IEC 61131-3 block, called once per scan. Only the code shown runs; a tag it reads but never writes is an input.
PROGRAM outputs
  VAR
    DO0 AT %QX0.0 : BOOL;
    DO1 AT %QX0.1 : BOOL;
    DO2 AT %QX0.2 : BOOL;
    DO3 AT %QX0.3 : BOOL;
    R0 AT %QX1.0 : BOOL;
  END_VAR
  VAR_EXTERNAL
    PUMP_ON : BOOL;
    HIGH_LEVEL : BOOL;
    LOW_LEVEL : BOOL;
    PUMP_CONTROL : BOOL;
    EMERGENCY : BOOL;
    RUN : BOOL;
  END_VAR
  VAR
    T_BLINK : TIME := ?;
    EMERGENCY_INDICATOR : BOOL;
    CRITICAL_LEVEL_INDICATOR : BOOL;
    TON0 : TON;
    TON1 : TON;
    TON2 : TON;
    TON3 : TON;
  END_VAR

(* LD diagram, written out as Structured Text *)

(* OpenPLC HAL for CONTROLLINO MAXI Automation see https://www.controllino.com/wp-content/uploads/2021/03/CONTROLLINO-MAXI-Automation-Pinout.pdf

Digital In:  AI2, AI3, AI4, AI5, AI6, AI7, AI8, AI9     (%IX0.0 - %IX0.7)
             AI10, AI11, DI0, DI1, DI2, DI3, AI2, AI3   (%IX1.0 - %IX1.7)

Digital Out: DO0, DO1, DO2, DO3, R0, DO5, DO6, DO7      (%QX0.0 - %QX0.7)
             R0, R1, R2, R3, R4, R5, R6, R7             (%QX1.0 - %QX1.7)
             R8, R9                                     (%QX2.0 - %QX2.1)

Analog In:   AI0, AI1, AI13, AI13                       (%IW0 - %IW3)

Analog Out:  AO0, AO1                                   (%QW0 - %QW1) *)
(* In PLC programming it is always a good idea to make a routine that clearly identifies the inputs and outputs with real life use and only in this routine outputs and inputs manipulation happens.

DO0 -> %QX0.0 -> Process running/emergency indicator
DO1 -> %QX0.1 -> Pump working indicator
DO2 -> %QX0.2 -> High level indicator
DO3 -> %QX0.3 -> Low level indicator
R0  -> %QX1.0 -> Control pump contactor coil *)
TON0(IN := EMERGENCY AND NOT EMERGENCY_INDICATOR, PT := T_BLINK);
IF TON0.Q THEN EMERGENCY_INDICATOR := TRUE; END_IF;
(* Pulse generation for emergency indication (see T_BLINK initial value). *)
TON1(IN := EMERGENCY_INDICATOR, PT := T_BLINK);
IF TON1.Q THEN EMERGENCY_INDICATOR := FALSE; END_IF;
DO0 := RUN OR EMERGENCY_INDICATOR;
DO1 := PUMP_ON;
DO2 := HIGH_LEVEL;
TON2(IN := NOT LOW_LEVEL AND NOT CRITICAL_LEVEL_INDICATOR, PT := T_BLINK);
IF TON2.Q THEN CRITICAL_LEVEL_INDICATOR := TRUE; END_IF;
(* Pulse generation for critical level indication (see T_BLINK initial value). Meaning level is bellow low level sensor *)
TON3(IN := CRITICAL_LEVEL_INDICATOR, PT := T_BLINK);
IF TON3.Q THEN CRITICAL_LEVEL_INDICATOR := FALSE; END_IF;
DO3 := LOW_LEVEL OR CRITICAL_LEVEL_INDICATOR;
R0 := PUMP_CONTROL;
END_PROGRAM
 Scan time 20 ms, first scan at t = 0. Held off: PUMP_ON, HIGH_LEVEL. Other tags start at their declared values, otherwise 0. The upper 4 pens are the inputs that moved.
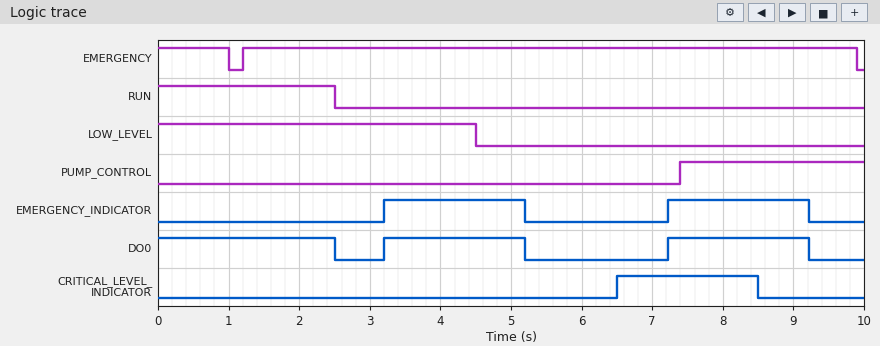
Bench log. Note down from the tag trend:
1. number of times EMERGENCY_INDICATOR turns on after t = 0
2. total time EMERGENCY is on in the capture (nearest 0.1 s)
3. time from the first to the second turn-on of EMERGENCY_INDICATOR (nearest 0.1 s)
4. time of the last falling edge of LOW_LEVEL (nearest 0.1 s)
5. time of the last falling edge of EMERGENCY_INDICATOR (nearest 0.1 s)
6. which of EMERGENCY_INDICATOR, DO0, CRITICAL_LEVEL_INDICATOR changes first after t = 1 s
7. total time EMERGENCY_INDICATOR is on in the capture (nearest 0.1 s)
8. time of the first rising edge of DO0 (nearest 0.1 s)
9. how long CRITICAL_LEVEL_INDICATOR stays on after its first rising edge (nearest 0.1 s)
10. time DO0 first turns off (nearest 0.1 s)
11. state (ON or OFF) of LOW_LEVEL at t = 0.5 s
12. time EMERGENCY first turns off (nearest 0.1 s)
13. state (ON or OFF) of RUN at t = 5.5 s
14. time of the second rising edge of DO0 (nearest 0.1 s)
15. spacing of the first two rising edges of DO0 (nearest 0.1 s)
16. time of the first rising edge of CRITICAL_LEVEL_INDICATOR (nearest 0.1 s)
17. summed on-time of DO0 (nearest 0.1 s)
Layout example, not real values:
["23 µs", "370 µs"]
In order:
["2", "9.7 s", "4.0 s", "4.5 s", "9.2 s", "DO0", "4.0 s", "3.2 s", "2.0 s", "2.5 s", "ON", "1.0 s", "OFF", "7.2 s", "4.0 s", "6.5 s", "6.5 s"]
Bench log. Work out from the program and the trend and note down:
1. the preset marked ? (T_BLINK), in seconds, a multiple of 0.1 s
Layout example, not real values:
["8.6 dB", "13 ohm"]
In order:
["2.0 s"]
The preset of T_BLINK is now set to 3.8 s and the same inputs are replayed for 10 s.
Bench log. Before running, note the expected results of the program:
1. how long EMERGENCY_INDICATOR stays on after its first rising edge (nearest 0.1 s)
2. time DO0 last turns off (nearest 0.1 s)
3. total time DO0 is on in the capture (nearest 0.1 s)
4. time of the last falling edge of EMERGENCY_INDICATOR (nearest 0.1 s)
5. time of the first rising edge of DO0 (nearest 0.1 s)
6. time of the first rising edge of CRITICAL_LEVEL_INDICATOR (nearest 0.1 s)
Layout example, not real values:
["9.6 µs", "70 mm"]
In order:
["3.8 s", "8.8 s", "6.3 s", "8.8 s", "5.0 s", "8.3 s"]
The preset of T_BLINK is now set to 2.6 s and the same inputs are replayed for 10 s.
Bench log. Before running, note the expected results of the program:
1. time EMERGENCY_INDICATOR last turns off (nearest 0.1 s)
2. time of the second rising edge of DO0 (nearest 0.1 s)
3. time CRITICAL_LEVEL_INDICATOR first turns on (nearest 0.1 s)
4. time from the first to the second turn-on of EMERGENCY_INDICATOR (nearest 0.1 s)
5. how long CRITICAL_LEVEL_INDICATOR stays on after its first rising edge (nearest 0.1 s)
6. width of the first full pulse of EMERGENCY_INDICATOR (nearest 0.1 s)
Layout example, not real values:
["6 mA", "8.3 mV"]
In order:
["6.4 s", "9.0 s", "7.1 s", "5.2 s", "2.6 s", "2.6 s"]
